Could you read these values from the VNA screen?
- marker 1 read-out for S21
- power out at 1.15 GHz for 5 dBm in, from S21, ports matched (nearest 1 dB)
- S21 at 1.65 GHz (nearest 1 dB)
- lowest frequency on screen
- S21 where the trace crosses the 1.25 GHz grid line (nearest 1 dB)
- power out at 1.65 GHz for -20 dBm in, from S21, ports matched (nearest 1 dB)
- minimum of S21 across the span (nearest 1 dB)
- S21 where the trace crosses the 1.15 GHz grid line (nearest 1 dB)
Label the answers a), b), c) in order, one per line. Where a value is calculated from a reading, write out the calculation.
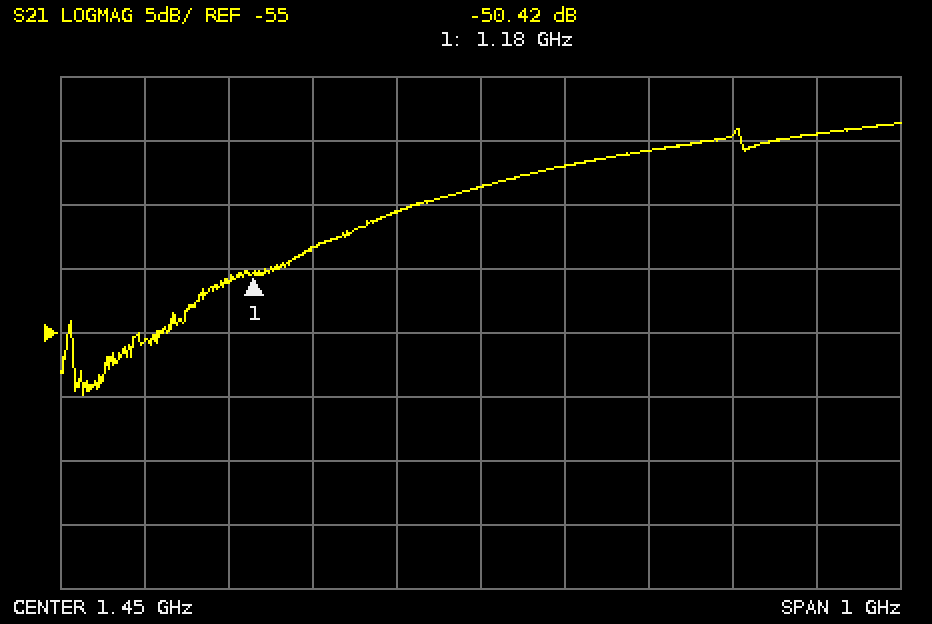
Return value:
a) -50.42 dB
b) 5 dBm + (-51 dB) = -46 dBm
c) -41 dB
d) 950 MHz
e) -48 dB
f) -20 dBm + (-41 dB) = -61 dBm
g) -60 dB
h) -51 dB
